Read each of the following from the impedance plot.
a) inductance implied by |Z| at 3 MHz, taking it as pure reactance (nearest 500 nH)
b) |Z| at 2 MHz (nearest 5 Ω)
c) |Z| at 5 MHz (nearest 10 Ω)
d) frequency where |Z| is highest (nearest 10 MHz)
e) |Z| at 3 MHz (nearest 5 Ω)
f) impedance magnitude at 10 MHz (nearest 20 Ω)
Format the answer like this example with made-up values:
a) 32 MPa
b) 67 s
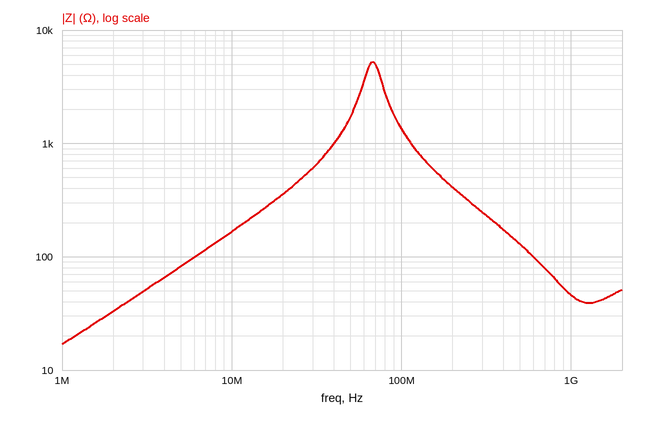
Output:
a) 2.5 µH
b) 35 Ω
c) 80 Ω
d) 70 MHz
e) 50 Ω
f) 160 Ω
